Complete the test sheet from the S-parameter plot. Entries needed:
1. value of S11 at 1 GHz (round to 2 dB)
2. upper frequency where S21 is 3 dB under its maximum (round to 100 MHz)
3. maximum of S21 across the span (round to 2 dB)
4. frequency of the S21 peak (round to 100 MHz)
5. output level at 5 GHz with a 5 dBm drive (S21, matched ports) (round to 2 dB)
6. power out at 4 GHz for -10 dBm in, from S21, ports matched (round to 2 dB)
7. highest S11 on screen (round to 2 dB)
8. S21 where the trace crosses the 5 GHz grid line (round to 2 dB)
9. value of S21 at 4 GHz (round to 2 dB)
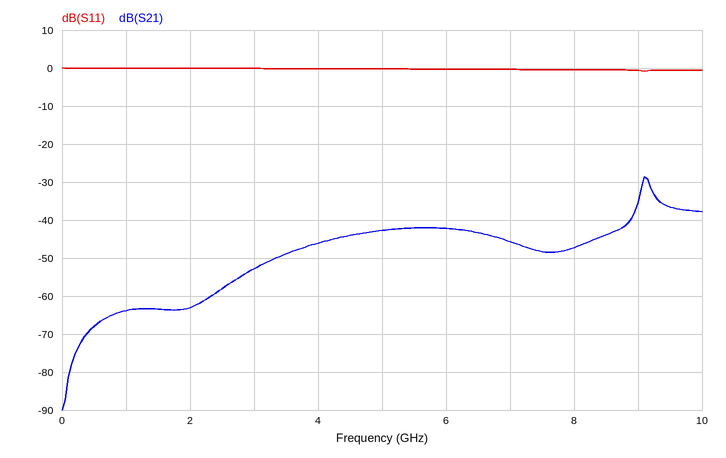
0 dB
9.2 GHz
-28 dB
9.1 GHz
-38 dBm
-56 dBm
0 dB
-42 dB
-46 dB
